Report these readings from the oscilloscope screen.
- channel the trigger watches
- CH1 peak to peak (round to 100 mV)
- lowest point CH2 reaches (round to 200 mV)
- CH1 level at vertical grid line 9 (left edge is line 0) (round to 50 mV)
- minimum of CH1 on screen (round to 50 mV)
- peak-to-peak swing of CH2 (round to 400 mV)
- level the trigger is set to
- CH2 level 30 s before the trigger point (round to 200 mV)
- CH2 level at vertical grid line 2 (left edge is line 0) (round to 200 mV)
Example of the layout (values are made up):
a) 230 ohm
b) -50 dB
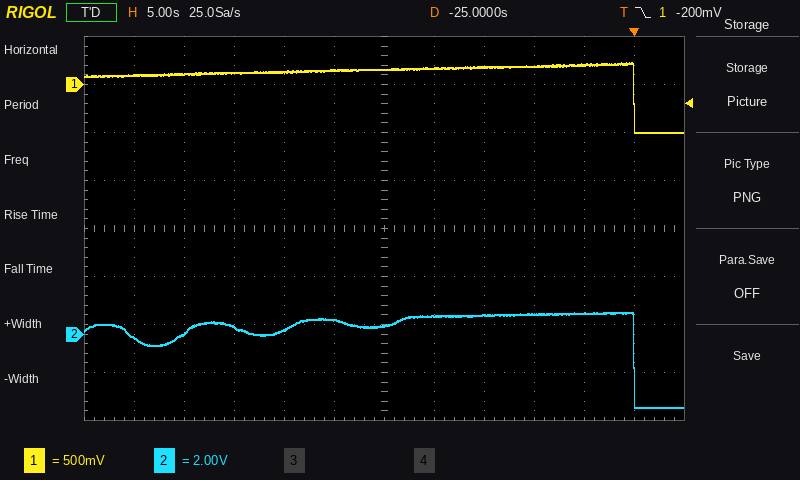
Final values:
a) CH1
b) 700 mV
c) -3.0 V
d) 200 mV
e) -500 mV
f) 4.0 V
g) -200 mV
h) 600 mV
i) 0.0 V
